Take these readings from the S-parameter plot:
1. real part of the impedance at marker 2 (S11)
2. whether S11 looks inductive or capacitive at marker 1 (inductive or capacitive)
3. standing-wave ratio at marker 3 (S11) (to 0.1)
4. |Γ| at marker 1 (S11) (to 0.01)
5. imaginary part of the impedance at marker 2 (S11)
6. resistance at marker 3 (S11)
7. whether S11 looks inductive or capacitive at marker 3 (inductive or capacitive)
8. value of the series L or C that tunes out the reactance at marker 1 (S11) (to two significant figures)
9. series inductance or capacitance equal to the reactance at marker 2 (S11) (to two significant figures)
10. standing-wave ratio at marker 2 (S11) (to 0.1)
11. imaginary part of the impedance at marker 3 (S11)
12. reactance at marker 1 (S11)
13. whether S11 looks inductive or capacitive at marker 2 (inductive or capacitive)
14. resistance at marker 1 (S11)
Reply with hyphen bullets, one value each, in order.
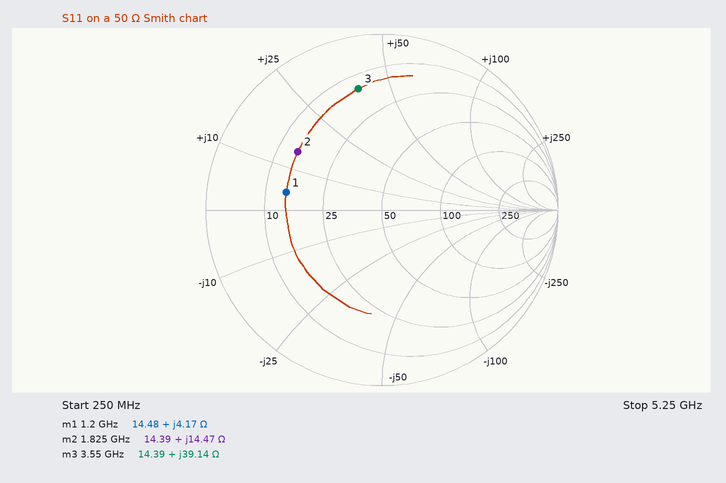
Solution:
- 14.39 Ω
- inductive
- 5.7
- 0.55
- +14.47 Ω
- 14.39 Ω
- inductive
- 32 pF
- 1.3 nH
- 3.8
- +39.14 Ω
- +4.17 Ω
- inductive
- 14.48 Ω
